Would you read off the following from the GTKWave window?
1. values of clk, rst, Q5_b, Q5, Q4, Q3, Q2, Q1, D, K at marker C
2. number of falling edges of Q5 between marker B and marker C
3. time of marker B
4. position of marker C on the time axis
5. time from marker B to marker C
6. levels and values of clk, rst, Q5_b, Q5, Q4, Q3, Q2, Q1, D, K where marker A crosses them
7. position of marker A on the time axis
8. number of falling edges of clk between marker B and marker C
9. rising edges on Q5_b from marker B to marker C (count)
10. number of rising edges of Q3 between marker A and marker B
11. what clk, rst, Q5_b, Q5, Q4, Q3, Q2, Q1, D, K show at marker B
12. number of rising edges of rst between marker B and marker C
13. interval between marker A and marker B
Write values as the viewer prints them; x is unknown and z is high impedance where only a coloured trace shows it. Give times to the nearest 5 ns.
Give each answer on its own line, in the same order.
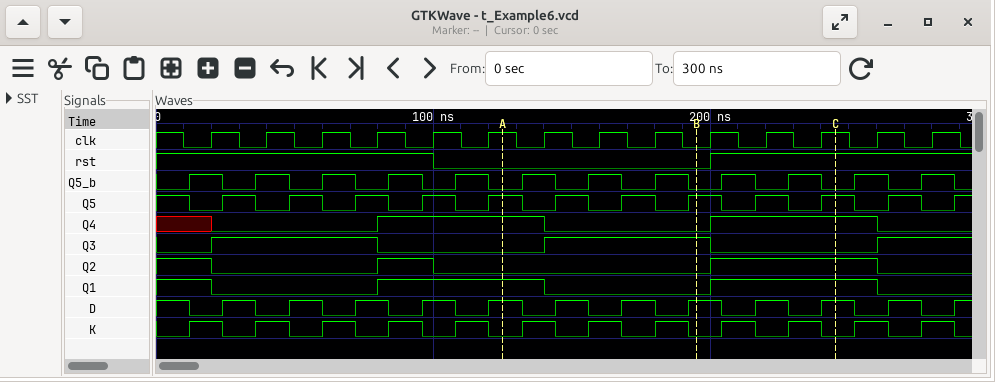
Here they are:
clk=1, rst=1, Q5_b=0, Q5=1, Q4=1, Q3=0, Q2=1, Q1=1, D=1, K=0
2
195 ns
245 ns
50 ns
clk=1, rst=0, Q5_b=0, Q5=1, Q4=1, Q3=0, Q2=0, Q1=1, D=1, K=0
125 ns
2
2
1
clk=0, rst=0, Q5_b=0, Q5=1, Q4=0, Q3=1, Q2=0, Q1=0, D=1, K=0
1
70 ns
